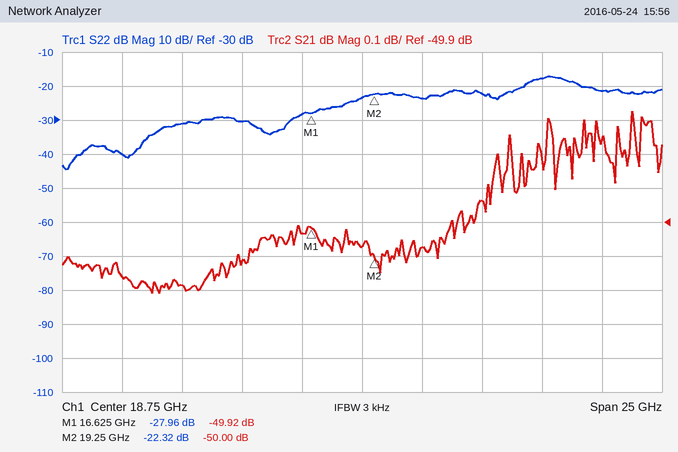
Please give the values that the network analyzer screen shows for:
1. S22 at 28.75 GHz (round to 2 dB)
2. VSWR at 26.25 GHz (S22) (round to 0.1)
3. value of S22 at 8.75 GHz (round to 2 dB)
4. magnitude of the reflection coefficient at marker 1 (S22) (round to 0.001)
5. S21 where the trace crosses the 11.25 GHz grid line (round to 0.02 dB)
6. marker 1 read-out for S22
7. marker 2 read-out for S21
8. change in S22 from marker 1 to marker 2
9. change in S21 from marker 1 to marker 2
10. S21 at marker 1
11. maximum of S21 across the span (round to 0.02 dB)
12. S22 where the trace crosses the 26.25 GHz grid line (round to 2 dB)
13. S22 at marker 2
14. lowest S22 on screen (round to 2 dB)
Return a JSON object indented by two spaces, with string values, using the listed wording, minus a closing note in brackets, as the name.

{
  "S22 at 28.75 GHz": "-22 dB",
  "VSWR at 26.25 GHz (S22)": "1.3",
  "value of S22 at 8.75 GHz": "-40 dB",
  "magnitude of the reflection coefficient at marker 1 (S22)": "0.040",
  "S21 where the trace crosses the 11.25 GHz grid line": "-50.08 dB",
  "marker 1 read-out for S22": "-27.96 dB",
  "marker 2 read-out for S21": "-50.00 dB",
  "change in S22 from marker 1 to marker 2": "5.64 dB",
  "change in S21 from marker 1 to marker 2": "-0.08 dB",
  "S21 at marker 1": "-49.92 dB",
  "maximum of S21 across the span": "-49.58 dB",
  "S22 where the trace crosses the 26.25 GHz grid line": "-18 dB",
  "S22 at marker 2": "-22.32 dB",
  "lowest S22 on screen": "-44 dB"
}
